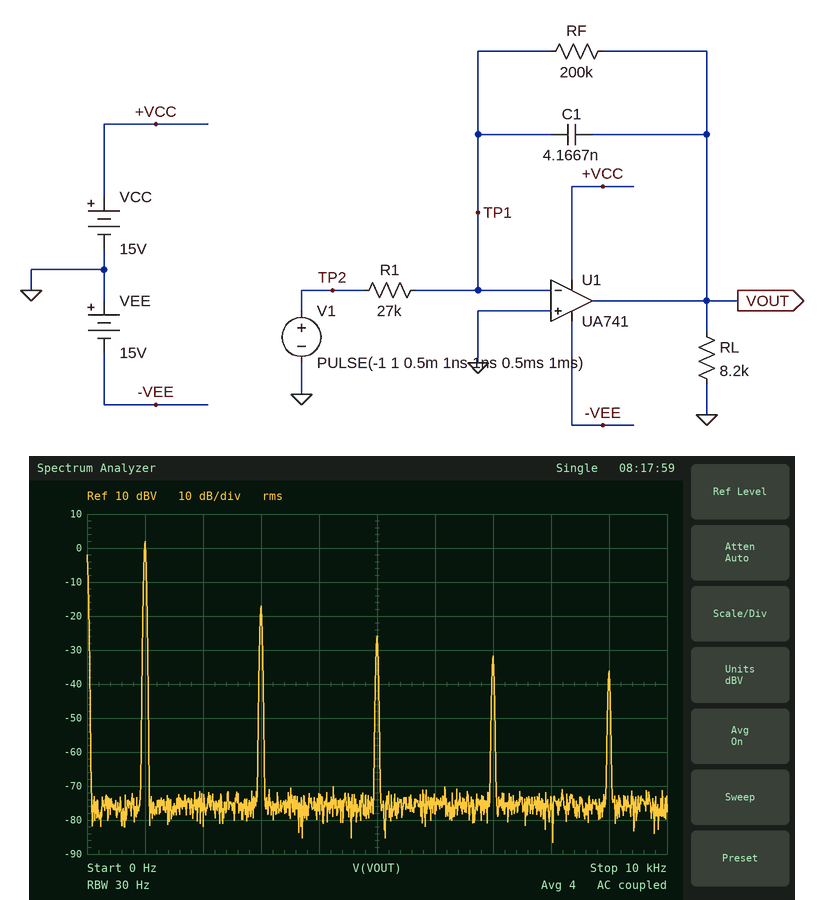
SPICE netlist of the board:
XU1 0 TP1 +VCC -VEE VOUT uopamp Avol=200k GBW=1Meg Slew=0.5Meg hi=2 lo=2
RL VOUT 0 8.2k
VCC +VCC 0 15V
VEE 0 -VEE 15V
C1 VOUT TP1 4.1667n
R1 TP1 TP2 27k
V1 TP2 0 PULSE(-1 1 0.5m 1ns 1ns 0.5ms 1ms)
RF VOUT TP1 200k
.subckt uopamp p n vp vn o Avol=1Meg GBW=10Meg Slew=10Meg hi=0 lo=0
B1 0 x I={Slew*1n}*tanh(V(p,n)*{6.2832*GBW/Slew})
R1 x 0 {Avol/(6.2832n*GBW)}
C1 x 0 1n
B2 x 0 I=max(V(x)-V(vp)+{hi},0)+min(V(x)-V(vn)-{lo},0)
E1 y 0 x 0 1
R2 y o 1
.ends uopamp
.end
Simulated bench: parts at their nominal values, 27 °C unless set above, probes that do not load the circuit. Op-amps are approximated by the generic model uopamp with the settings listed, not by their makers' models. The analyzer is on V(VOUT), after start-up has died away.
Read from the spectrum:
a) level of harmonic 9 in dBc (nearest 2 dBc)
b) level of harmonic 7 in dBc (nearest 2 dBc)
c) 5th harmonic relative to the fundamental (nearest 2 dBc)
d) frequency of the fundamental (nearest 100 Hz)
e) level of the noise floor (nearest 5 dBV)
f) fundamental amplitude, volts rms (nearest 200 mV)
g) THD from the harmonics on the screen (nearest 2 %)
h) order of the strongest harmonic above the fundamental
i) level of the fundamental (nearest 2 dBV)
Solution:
-38 dBc
-34 dBc
-28 dBc
1.0 kHz
-75 dBV
1.2 V
12 %
3
2 dBV
